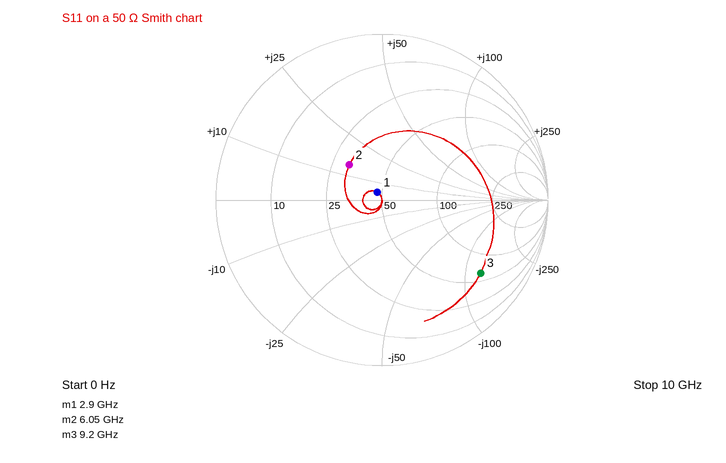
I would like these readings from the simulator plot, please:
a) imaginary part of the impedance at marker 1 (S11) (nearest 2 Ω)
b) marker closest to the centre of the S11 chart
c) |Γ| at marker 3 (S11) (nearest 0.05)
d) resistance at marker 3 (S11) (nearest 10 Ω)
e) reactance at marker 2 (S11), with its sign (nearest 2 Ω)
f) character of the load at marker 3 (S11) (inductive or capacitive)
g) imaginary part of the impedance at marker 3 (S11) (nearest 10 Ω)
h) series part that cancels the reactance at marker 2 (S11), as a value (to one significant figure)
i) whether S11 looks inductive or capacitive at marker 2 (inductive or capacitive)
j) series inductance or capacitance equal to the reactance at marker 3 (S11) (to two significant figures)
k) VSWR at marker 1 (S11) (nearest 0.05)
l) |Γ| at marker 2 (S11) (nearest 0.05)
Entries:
+4 Ω
marker 1
0.75
60 Ω
+14 Ω
capacitive
-120 Ω
2 pF
inductive
140 fF
1.10
0.30
